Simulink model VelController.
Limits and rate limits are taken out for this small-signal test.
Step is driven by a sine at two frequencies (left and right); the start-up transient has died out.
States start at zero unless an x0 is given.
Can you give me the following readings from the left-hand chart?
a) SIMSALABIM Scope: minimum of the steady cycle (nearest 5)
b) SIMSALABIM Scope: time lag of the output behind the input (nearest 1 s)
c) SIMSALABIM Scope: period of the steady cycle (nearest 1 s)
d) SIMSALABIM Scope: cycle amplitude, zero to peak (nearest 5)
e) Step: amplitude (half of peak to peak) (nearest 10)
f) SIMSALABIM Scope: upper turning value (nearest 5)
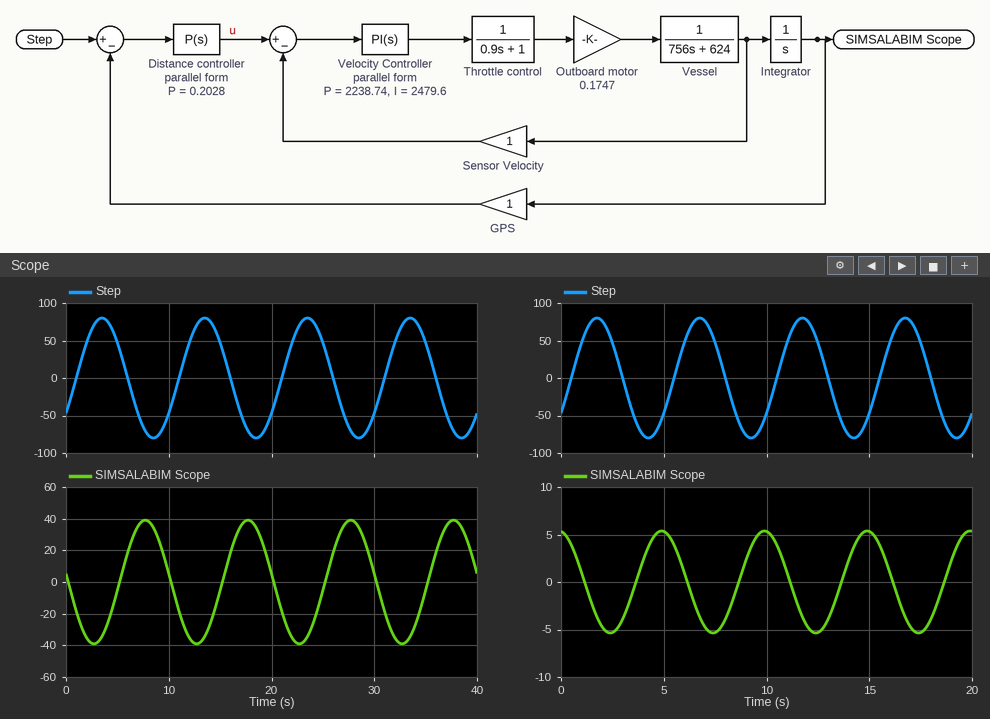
-40
4 s
10 s
40
80
40
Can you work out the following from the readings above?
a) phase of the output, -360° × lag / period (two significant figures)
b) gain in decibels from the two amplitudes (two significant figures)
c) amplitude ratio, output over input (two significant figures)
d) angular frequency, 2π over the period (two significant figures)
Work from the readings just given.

-140°
-6.0 dB
0.50
0.63 rad/s
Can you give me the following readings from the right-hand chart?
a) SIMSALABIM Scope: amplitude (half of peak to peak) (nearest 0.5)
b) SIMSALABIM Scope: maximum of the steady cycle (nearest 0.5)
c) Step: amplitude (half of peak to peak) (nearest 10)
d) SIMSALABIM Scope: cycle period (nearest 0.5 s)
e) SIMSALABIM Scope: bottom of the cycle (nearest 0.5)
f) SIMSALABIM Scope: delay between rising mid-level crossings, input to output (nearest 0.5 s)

5.5
5.5
80
5.0 s
-5.5
3.0 s
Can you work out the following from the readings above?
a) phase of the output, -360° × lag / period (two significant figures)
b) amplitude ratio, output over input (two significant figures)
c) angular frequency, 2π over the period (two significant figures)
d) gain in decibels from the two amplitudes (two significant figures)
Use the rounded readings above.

-220°
0.069
1.3 rad/s
-23 dB
